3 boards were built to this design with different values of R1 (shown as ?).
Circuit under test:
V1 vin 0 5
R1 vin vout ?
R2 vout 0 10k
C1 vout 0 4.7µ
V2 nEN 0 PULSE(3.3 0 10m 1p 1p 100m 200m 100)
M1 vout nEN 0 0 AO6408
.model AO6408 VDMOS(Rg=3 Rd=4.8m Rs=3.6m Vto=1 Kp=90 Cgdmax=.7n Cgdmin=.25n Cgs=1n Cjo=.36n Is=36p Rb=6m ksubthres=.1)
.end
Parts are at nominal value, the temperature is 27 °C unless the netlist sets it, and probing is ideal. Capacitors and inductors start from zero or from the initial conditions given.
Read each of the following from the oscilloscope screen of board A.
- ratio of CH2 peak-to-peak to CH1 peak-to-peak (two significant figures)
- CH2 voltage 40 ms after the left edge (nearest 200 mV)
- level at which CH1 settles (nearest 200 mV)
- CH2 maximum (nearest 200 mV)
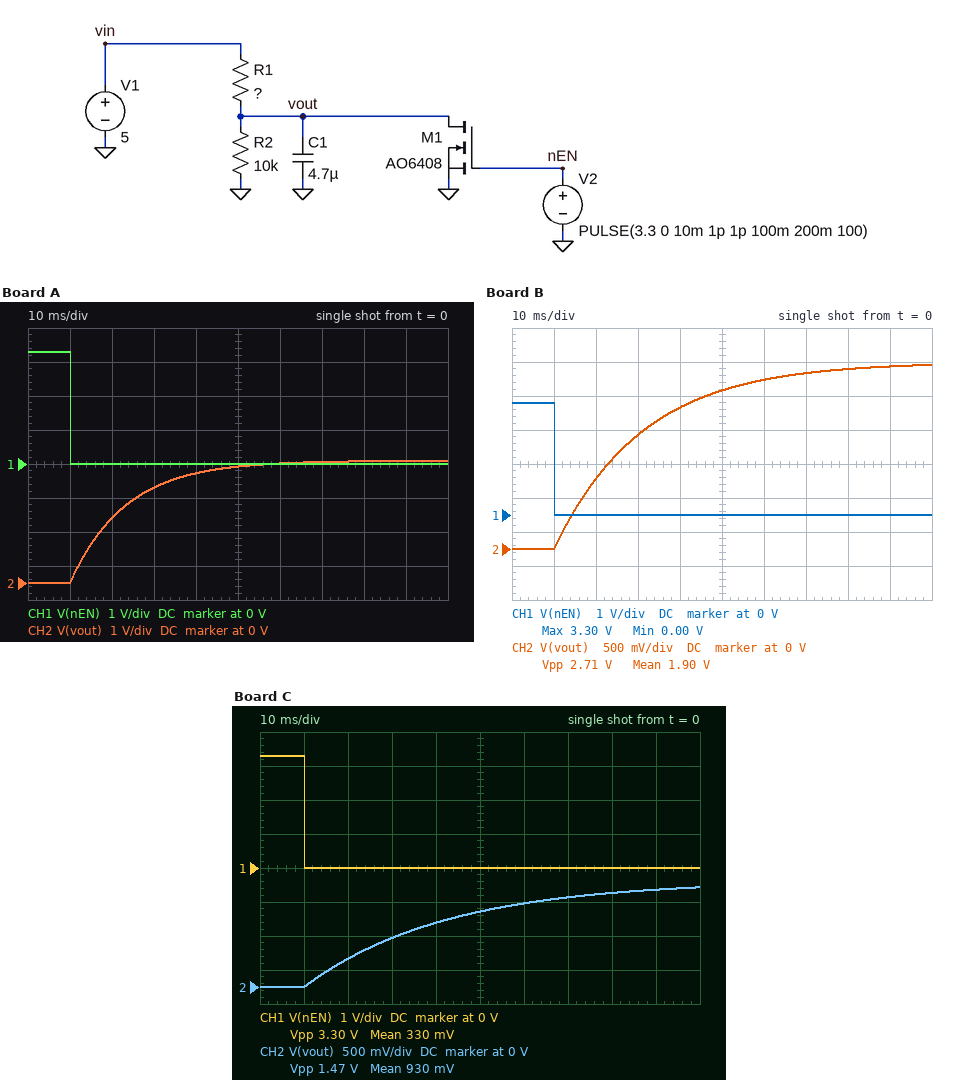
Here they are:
1.1
3.2 V
0 V
3.6 V
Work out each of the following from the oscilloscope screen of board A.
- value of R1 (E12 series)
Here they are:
3.9 kΩ
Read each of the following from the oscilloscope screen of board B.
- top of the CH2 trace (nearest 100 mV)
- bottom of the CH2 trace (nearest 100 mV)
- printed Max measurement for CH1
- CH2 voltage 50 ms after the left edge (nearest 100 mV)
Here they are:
2.7 V
0 V
3.30 V
2.3 V
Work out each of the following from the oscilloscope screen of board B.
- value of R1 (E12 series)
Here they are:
8.2 kΩ
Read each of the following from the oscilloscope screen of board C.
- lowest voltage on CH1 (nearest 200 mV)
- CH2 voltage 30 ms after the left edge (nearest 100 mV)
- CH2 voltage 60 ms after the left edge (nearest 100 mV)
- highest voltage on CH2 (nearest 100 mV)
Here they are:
0 V
700 mV
1.2 V
1.5 V
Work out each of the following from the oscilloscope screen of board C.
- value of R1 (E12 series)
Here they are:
22 kΩ
